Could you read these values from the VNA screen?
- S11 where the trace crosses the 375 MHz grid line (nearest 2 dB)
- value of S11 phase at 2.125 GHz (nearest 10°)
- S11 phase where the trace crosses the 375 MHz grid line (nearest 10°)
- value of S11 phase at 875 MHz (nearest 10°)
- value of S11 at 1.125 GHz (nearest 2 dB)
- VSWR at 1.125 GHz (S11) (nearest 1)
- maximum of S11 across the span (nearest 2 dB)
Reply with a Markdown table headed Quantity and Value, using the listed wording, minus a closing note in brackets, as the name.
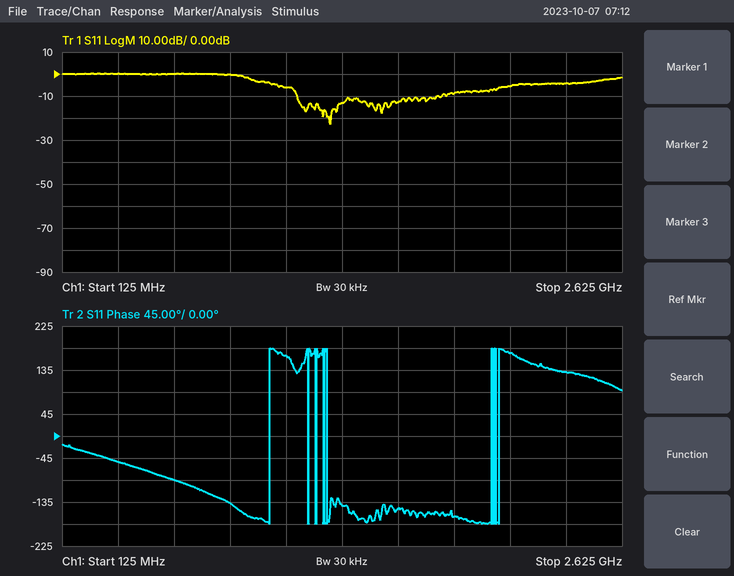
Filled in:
| Quantity | Value |
|---|---|
| S11 where the trace crosses the 375 MHz grid line | 0 dB |
| value of S11 phase at 2.125 GHz | 170° |
| S11 phase where the trace crosses the 375 MHz grid line | -50° |
| value of S11 phase at 875 MHz | -140° |
| value of S11 at 1.125 GHz | -6 dB |
| VSWR at 1.125 GHz (S11) | 3 |
| maximum of S11 across the span | 0 dB |
